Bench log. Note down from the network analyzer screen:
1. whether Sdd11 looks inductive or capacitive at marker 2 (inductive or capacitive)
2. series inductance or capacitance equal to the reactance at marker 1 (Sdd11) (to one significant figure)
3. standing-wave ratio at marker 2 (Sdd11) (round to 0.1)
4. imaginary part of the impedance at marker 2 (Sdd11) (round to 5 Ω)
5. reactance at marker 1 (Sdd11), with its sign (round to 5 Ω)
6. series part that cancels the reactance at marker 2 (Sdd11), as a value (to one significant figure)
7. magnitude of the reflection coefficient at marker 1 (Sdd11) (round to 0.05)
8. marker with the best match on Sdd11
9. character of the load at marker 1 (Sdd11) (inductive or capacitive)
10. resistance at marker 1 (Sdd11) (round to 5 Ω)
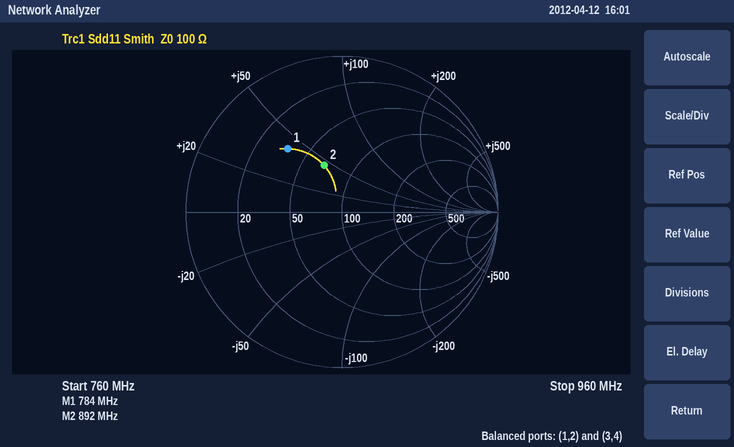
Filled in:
inductive
8 nH
1.9
+45 Ω
+40 Ω
4 pF
0.55
marker 2
inductive
35 Ω
